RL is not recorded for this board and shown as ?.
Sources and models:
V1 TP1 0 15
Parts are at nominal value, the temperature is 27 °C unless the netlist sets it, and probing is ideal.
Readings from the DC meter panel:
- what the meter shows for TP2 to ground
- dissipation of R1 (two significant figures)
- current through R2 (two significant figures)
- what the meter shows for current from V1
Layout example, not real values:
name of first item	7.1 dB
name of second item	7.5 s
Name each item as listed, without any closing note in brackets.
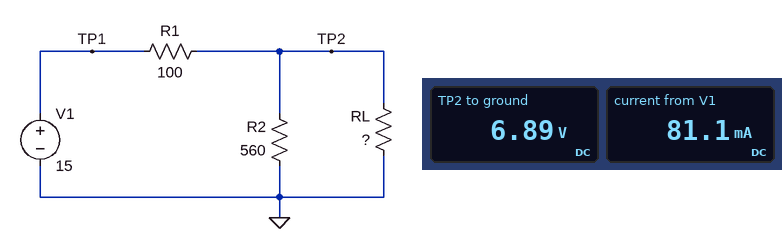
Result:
what the meter shows for TP2 to ground	6.89 V
dissipation of R1	660 mW
current through R2	12 mA
what the meter shows for current from V1	81.1 mA
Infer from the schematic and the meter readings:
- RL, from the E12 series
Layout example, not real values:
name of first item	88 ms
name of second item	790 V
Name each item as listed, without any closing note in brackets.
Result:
RL, from the E12 series	100 Ω
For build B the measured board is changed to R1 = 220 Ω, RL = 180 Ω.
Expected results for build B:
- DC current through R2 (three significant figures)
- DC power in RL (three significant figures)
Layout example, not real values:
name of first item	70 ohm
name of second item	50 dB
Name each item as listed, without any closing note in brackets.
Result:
DC current through R2	10.2 mA
DC power in RL	183 mW
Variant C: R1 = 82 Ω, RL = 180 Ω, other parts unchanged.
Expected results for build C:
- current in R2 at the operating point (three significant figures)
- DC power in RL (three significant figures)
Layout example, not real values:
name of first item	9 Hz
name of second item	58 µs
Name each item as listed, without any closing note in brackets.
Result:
current in R2 at the operating point	16.7 mA
DC power in RL	487 mW
